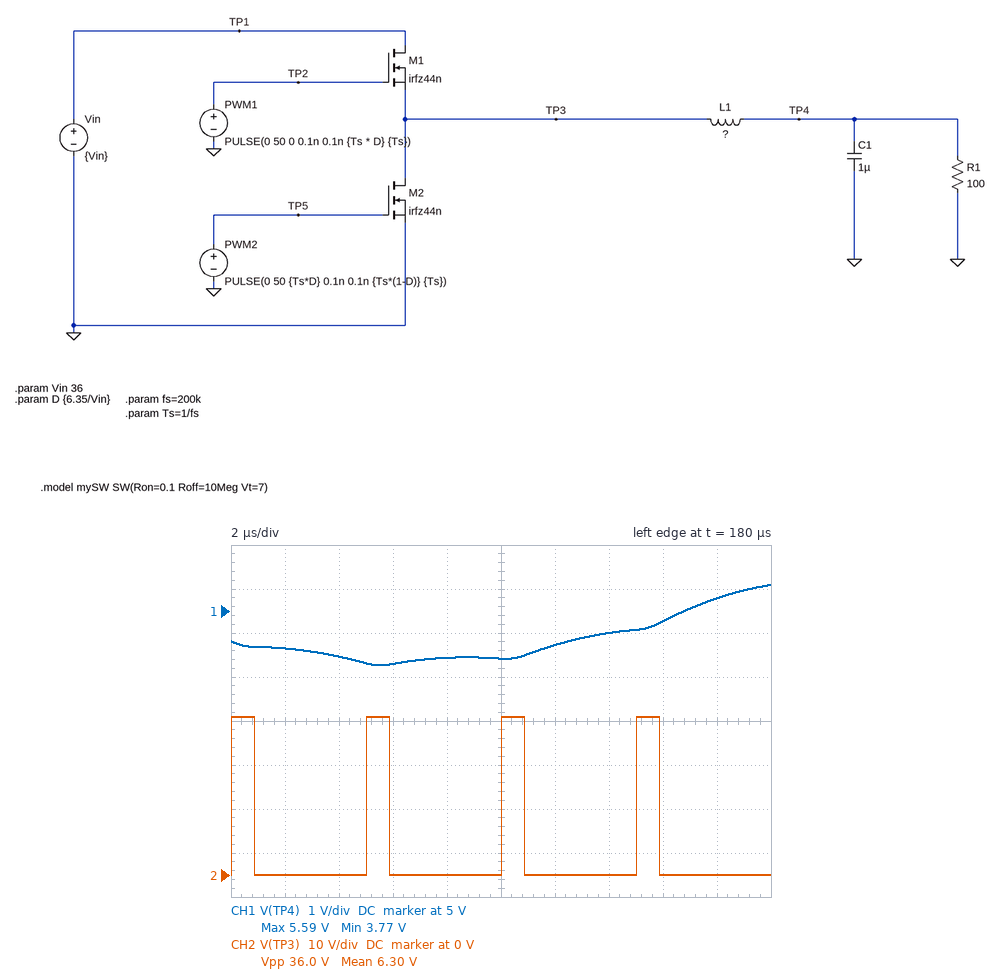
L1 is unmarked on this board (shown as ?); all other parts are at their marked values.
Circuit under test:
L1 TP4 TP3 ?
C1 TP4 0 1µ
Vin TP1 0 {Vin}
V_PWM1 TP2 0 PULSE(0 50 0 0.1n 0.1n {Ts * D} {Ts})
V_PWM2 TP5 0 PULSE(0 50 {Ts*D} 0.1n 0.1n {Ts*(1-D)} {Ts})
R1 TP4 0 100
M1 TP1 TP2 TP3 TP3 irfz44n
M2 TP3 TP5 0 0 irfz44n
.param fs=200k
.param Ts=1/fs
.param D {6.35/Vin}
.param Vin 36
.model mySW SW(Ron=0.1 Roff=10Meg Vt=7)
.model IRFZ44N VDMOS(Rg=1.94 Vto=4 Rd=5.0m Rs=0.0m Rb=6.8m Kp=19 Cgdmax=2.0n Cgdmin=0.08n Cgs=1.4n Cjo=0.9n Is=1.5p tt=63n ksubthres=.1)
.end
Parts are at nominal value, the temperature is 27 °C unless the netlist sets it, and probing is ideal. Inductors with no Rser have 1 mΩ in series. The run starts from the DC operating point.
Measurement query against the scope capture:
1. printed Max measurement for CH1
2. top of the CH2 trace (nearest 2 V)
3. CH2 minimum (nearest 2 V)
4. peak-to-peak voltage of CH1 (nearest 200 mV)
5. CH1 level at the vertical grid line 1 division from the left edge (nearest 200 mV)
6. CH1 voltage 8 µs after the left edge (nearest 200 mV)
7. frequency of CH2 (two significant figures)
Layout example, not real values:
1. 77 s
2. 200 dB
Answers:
1. 5.59 V
2. 36 V
3. 0 V
4. 1.8 V
5. 4.2 V
6. 4.0 V
7. 200 kHz
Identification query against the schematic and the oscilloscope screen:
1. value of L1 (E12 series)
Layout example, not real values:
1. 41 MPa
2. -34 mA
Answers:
1. 100 µH
